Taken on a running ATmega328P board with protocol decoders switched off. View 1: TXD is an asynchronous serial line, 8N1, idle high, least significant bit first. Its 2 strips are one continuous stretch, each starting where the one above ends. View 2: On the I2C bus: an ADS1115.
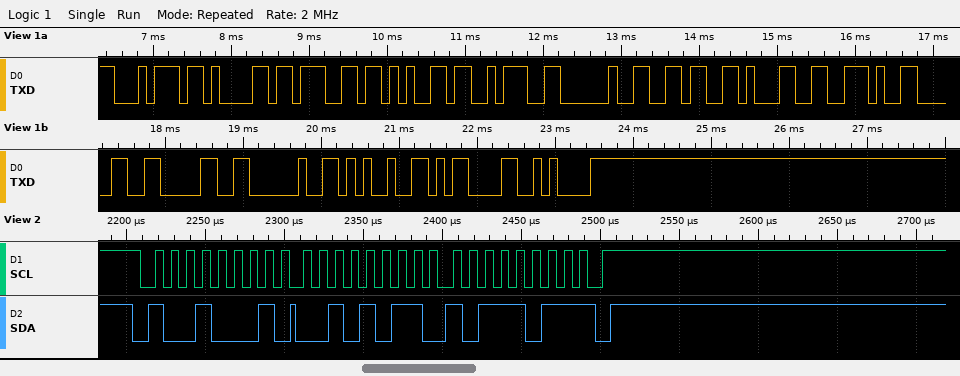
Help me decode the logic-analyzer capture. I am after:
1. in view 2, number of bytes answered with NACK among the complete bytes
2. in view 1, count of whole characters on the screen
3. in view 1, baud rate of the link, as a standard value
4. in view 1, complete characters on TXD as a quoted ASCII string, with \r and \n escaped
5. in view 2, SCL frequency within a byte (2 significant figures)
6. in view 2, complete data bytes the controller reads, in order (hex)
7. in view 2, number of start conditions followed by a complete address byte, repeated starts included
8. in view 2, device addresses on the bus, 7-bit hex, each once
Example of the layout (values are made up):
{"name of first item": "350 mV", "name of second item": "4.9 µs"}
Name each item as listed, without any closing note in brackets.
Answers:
{"in view 2, number of bytes answered with NACK among the complete bytes": "1", "in view 1, count of whole characters on the screen": "15", "in view 1, baud rate of the link, as a standard value": "9600 baud", "in view 1, complete characters on TXD as a quoted ASCII string, with \\r and \\n escaped": "\"tage: 61.00 %\\r\\n\"", "in view 2, SCL frequency within a byte": "100 kHz", "in view 2, complete data bytes the controller reads, in order": "2B BB", "in view 2, number of start conditions followed by a complete address byte, repeated starts included": "1", "in view 2, device addresses on the bus, 7-bit hex, each once": "0x48"}
